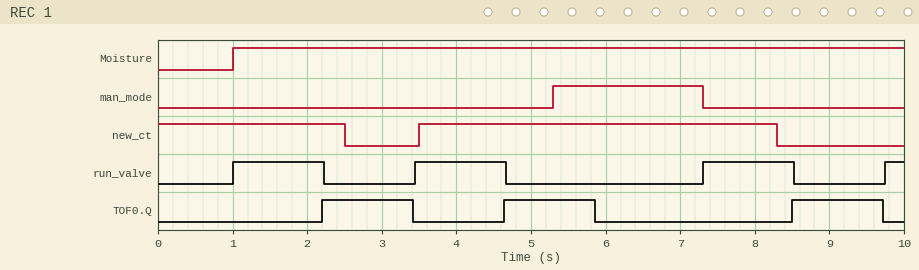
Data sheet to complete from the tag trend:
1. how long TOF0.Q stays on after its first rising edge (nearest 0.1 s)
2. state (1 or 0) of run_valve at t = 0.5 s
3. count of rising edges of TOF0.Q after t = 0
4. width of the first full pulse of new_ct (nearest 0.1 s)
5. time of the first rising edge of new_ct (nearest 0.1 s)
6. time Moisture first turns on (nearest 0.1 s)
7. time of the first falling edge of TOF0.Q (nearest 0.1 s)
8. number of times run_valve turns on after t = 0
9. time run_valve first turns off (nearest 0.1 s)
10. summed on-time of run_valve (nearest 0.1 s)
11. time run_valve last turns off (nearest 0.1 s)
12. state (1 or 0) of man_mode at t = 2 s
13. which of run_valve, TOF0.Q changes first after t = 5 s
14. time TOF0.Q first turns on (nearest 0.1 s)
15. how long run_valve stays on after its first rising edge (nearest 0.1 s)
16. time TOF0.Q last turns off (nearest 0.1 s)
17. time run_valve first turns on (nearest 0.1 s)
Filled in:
1.2 s
0
3
4.8 s
3.5 s
1.0 s
3.4 s
4
2.2 s
3.9 s
8.5 s
0
TOF0.Q
2.2 s
1.2 s
9.7 s
1.0 s
